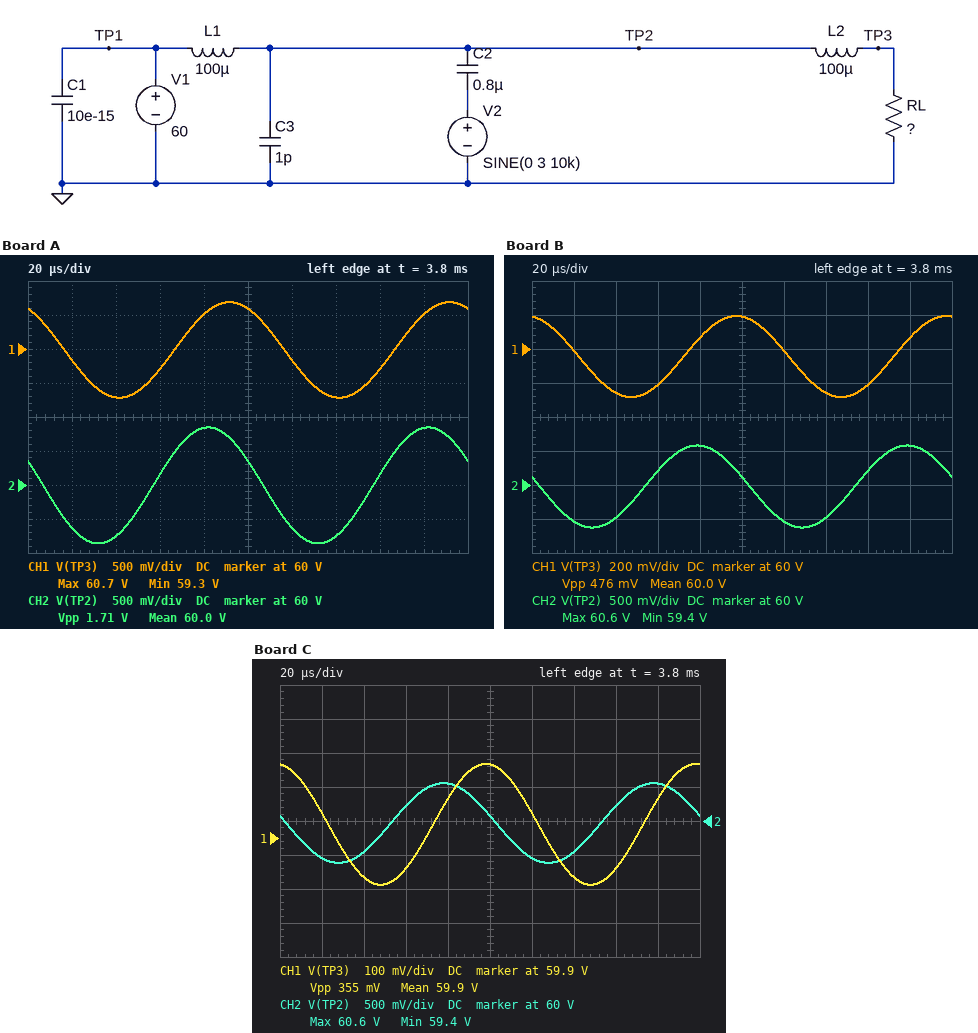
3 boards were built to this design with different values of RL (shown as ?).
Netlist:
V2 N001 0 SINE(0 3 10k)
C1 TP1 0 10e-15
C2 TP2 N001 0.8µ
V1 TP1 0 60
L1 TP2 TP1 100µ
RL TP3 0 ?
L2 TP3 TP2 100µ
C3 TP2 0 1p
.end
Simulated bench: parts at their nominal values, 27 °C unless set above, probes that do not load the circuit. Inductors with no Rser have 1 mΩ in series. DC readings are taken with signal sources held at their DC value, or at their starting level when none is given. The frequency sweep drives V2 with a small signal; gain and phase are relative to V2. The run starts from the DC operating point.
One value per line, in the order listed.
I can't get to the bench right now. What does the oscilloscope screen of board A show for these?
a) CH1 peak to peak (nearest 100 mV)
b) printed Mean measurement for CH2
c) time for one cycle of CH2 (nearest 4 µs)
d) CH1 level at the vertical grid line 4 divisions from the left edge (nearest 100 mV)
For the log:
1.4 V
60.0 V
100 µs
60.5 V
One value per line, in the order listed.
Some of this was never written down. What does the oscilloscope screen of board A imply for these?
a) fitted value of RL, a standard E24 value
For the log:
9.1 Ω
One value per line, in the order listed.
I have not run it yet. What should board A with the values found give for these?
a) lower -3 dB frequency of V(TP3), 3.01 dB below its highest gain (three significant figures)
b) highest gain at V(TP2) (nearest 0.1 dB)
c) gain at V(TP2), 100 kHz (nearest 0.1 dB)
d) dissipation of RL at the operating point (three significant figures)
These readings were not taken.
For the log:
21.1 kHz
12.2 dB
0.6 dB
395 W
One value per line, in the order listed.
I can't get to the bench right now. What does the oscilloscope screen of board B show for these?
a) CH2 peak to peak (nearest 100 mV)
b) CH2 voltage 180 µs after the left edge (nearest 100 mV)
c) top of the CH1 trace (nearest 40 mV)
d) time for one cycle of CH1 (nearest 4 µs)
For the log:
1.2 V
60.6 V
60.20 V
100 µs
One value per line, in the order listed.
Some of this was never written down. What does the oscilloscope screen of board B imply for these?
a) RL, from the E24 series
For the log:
2.7 Ω
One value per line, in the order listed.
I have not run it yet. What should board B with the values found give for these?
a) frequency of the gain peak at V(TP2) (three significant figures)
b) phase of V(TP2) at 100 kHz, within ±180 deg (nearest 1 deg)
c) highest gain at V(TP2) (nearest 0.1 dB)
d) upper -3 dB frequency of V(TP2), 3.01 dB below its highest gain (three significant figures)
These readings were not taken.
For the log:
25.1 kHz
0 deg
21.5 dB
26.3 kHz
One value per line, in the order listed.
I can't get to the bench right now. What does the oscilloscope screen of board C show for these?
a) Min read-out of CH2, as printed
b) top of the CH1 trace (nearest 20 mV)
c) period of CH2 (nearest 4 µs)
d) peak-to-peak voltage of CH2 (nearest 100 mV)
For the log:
59.4 V
60.12 V
100 µs
1.2 V
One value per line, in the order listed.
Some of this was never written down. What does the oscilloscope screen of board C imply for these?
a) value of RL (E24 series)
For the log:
2 Ω
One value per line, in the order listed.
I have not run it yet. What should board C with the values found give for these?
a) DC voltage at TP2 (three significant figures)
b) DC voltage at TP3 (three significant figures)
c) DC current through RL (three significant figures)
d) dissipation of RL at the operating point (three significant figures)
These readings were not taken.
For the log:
60.0 V
59.9 V
30.0 A
1.80 kW
